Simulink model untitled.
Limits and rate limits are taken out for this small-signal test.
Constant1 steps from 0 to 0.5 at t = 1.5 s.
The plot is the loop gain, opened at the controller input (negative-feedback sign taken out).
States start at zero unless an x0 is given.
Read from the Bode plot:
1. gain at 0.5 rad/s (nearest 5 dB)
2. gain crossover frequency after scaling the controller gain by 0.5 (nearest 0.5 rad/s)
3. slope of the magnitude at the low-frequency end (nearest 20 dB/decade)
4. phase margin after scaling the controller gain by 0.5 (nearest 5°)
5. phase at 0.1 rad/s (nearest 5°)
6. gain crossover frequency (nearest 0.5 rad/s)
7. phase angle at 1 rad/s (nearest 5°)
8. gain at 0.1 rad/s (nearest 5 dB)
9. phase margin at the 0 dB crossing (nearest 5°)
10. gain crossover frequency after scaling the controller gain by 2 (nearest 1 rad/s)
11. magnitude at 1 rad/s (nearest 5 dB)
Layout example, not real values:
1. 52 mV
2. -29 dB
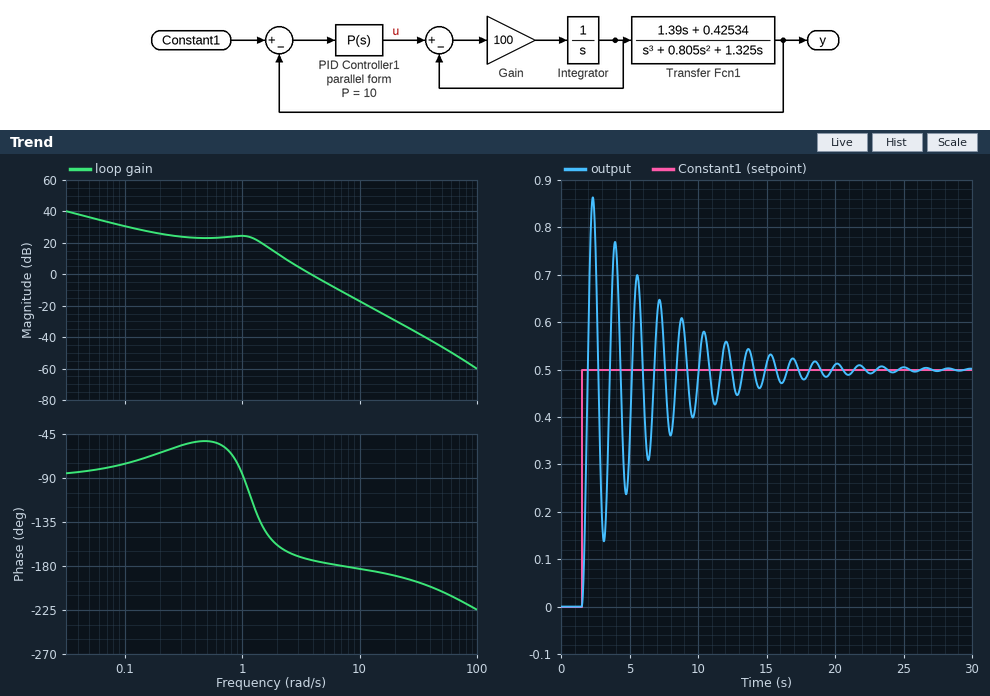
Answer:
1. 25 dB
2. 3.0 rad/s
3. -20 dB/decade
4. 10°
5. -75°
6. 4.0 rad/s
7. -85°
8. 30 dB
9. 5°
10. 5 rad/s
11. 25 dB
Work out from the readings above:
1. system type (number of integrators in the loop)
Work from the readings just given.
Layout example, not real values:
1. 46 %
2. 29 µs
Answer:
1. 1
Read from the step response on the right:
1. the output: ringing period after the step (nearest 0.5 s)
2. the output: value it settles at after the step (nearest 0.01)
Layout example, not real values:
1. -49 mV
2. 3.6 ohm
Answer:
1. 1.5 s
2. 0.50
